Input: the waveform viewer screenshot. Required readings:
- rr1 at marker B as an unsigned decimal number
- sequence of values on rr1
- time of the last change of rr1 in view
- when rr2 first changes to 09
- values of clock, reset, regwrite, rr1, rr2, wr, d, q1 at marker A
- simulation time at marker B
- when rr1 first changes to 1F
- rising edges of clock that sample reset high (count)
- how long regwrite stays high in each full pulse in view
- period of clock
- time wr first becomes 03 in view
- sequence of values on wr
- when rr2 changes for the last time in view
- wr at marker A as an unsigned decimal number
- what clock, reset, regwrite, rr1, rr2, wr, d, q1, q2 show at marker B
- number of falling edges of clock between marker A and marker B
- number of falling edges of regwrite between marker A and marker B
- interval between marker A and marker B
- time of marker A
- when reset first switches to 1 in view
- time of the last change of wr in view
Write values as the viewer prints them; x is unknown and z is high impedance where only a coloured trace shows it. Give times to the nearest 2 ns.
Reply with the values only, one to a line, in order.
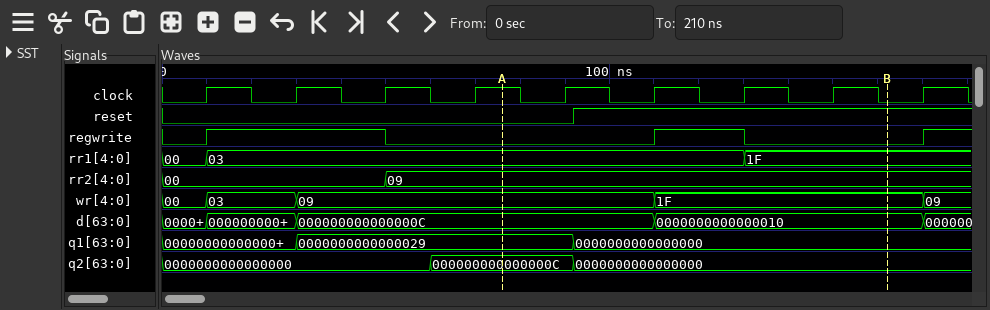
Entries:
31
00, 03, 1F
130 ns
50 ns
clock=1, reset=0, regwrite=0, rr1=03, rr2=09, wr=09, d=000000000000000C, q1=0000000000000029
162 ns
130 ns
4
40 ns, 20 ns
20 ns
10 ns
00, 03, 09, 1F, 09
50 ns
9
clock=0, reset=1, regwrite=0, rr1=1F, rr2=09, wr=1F, d=0000000000000010, q1=0000000000000000, q2=0000000000000000
5
1
86 ns
76 ns
92 ns
170 ns
